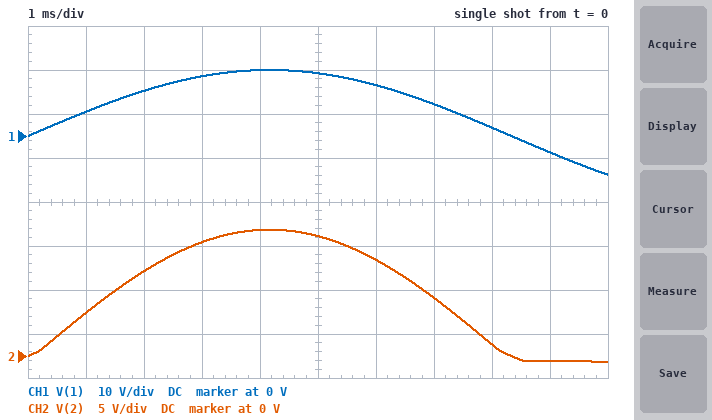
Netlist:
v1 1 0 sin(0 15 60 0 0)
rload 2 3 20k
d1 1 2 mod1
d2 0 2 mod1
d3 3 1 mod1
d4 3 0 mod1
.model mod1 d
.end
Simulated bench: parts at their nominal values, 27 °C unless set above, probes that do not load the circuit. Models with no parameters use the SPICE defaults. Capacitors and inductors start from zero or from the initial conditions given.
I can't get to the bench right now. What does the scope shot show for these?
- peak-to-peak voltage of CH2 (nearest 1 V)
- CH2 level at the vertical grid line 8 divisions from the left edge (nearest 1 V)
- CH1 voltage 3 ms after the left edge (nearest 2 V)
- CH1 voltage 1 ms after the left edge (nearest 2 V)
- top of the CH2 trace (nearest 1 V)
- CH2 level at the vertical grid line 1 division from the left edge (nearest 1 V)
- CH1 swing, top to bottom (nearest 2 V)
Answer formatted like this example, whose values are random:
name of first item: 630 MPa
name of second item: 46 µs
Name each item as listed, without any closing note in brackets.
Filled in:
peak-to-peak voltage of CH2: 15 V
CH2 level at the vertical grid line 8 divisions from the left edge: 1 V
CH1 voltage 3 ms after the left edge: 14 V
CH1 voltage 1 ms after the left edge: 6 V
top of the CH2 trace: 14 V
CH2 level at the vertical grid line 1 division from the left edge: 5 V
CH1 swing, top to bottom: 24 V
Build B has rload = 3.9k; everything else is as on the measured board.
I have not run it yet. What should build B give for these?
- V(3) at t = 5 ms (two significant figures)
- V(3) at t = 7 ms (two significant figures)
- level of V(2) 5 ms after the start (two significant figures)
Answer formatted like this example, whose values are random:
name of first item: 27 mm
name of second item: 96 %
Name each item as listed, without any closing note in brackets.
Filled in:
V(3) at t = 5 ms: 690 mV
V(3) at t = 7 ms: 670 mV
level of V(2) 5 ms after the start: 14 V
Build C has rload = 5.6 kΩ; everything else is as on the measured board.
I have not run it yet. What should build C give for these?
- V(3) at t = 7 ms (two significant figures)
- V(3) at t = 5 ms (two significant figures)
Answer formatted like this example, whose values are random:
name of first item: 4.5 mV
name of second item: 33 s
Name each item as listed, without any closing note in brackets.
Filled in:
V(3) at t = 7 ms: 660 mV
V(3) at t = 5 ms: 680 mV
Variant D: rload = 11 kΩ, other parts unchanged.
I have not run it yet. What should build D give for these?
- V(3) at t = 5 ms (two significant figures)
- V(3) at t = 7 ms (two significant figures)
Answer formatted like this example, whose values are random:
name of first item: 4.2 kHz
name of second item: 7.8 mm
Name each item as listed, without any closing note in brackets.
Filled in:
V(3) at t = 5 ms: 660 mV
V(3) at t = 7 ms: 640 mV
